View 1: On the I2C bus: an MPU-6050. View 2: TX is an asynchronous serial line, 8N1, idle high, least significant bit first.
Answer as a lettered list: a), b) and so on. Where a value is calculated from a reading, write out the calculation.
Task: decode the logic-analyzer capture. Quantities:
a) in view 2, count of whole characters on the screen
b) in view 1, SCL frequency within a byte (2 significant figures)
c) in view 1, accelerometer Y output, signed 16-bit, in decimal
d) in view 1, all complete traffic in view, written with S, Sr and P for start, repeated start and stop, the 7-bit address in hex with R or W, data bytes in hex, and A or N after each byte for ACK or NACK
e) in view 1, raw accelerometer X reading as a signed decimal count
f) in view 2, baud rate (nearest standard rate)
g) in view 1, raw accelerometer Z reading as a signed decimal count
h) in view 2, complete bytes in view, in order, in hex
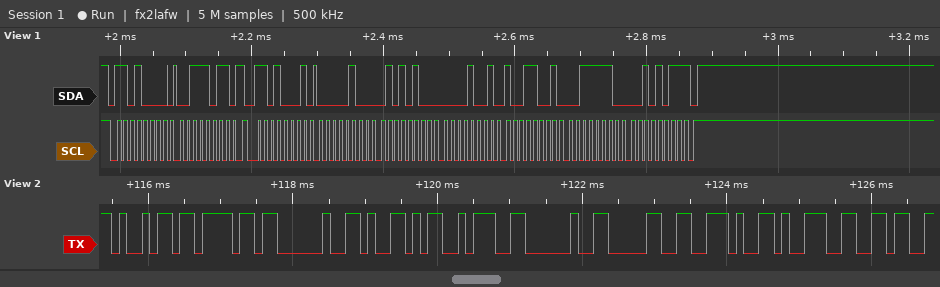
a) 10
b) 100 kHz
c) 0x0999 = 2457
d) S 68W A 3B A Sr 68R A 04 A 54 A 09 A 99 A 3E A 2B N P
e) 0x0454 = 1108
f) 9600 baud
g) 0x3E2B = 15915
h) 0x69 0x6F 0x20 0x59 0x3A 0x20 0x30 0x2E 0x39 0x36
